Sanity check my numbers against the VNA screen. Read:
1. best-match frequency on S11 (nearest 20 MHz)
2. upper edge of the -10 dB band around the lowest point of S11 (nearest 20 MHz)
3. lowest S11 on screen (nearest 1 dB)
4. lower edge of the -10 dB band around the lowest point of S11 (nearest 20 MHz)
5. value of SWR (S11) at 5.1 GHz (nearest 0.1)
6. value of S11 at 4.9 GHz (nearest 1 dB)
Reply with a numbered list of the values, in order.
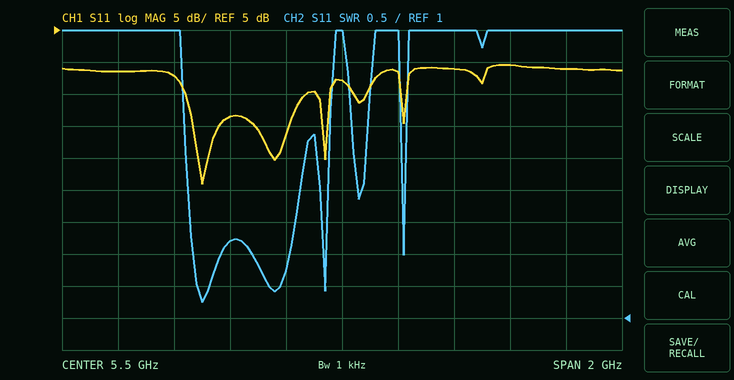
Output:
1. 5.00 GHz
2. 5.06 GHz
3. -19 dB
4. 4.96 GHz
5. 2.2
6. -2 dB
